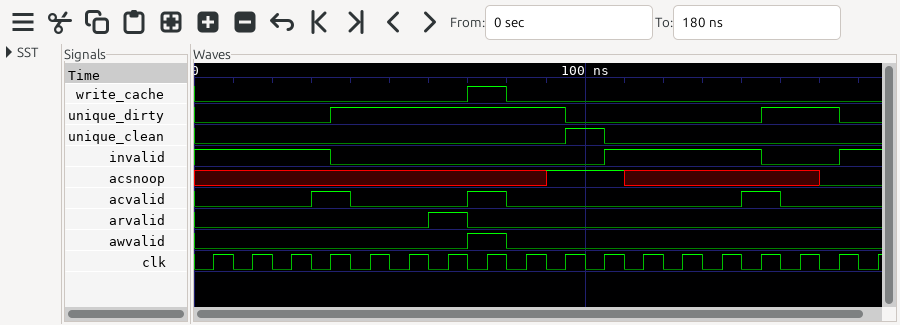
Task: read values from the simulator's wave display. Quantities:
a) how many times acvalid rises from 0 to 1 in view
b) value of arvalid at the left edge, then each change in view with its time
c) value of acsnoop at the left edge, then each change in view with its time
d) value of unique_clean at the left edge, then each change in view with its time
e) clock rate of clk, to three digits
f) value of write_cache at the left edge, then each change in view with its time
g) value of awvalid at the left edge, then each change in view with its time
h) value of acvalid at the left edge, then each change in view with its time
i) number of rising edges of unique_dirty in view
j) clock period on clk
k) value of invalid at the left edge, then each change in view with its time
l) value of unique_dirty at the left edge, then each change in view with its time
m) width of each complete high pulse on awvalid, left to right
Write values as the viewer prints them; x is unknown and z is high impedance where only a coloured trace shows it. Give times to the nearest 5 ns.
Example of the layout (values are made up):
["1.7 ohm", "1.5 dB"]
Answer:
["3", "0, 1 at 60 ns, 0 at 70 ns", "x, 1 at 90 ns, x at 110 ns, 0 at 160 ns", "0, 1 at 95 ns, 0 at 105 ns", "100 MHz", "0, 1 at 70 ns, 0 at 80 ns", "0, 1 at 70 ns, 0 at 80 ns", "0, 1 at 30 ns, 0 at 40 ns, 1 at 70 ns, 0 at 80 ns, 1 at 140 ns, 0 at 150 ns", "2", "10 ns", "1, 0 at 35 ns, 1 at 105 ns, 0 at 145 ns, 1 at 165 ns", "0, 1 at 35 ns, 0 at 95 ns, 1 at 145 ns, 0 at 165 ns", "10 ns"]
